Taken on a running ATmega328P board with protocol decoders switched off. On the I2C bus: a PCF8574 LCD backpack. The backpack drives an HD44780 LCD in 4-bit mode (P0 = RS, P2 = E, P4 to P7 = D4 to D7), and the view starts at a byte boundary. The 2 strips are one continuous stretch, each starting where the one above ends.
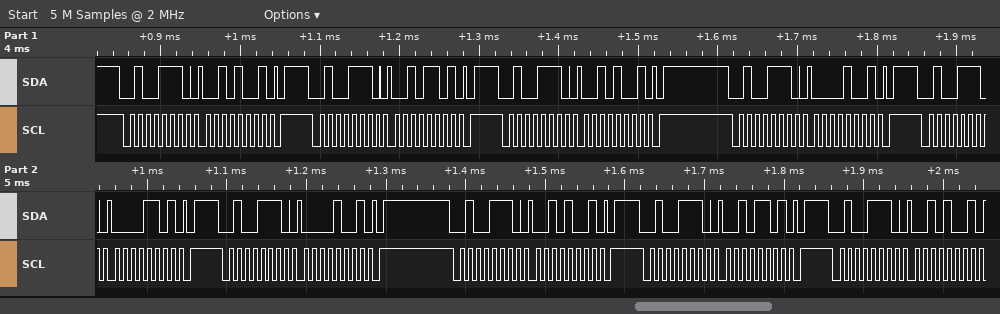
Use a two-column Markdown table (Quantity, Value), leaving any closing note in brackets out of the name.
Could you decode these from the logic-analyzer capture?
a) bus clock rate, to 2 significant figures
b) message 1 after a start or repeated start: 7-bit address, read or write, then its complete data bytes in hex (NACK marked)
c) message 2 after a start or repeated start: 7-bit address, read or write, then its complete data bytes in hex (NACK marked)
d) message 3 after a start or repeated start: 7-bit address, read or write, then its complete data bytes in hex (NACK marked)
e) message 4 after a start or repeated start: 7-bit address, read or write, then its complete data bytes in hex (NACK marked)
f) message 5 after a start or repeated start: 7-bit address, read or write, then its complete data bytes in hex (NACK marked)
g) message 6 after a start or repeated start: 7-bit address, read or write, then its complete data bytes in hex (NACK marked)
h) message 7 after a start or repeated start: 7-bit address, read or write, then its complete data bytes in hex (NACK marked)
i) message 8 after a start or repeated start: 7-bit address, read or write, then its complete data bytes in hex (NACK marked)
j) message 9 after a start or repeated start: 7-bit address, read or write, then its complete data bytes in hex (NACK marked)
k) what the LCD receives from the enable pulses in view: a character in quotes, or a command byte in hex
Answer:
| Quantity | Value |
|---|---|
| bus clock rate, to 2 significant figures | 100 kHz |
| message 1 after a start or repeated start: 7-bit address, read or write, then its complete data bytes in hex | 0x27 write: 29 |
| message 2 after a start or repeated start: 7-bit address, read or write, then its complete data bytes in hex | 0x27 write: 2D |
| message 3 after a start or repeated start: 7-bit address, read or write, then its complete data bytes in hex | 0x27 write: 29 |
| message 4 after a start or repeated start: 7-bit address, read or write, then its complete data bytes in hex | 0x27 write: 09 |
| message 5 after a start or repeated start: 7-bit address, read or write, then its complete data bytes in hex | 0x27 write: 0D |
| message 6 after a start or repeated start: 7-bit address, read or write, then its complete data bytes in hex | 0x27 write: 09 |
| message 7 after a start or repeated start: 7-bit address, read or write, then its complete data bytes in hex | 0x27 write: 29 |
| message 8 after a start or repeated start: 7-bit address, read or write, then its complete data bytes in hex | 0x27 write: 2D |
| message 9 after a start or repeated start: 7-bit address, read or write, then its complete data bytes in hex | 0x27 write: 29 |
| what the LCD receives from the enable pulses in view: a character in quotes, or a command byte in hex | ' ' |
